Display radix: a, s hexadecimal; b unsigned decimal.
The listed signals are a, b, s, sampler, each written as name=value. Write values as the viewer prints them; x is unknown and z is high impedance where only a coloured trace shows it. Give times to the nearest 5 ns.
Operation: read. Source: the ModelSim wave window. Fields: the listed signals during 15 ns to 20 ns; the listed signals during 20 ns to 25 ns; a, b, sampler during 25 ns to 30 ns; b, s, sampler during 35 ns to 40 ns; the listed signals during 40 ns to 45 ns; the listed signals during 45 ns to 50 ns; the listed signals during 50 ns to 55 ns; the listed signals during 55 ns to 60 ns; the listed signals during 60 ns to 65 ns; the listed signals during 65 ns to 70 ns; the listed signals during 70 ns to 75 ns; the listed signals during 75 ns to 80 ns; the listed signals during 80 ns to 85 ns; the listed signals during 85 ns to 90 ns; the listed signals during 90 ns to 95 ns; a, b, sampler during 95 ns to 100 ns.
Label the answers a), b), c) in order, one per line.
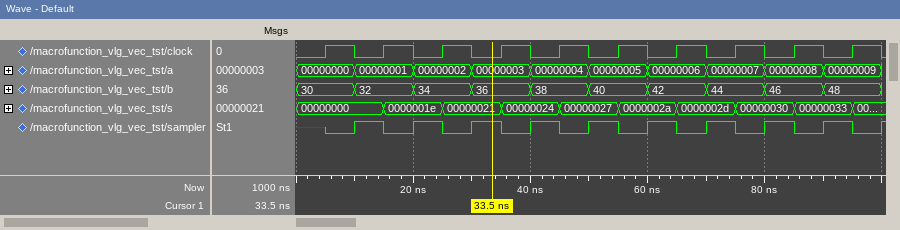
a) a=00000001, b=32, s=0000001e, sampler=0
b) a=00000002, b=34, s=0000001e, sampler=1
c) a=00000002, b=34, sampler=0
d) b=36, s=00000024, sampler=0
e) a=00000004, b=38, s=00000024, sampler=1
f) a=00000004, b=38, s=00000027, sampler=0
g) a=00000005, b=40, s=00000027, sampler=1
h) a=00000005, b=40, s=0000002a, sampler=0
i) a=00000006, b=42, s=0000002a, sampler=1
j) a=00000006, b=42, s=0000002d, sampler=0
k) a=00000007, b=44, s=0000002d, sampler=1
l) a=00000007, b=44, s=00000030, sampler=0
m) a=00000008, b=46, s=00000030, sampler=1
n) a=00000008, b=46, s=00000033, sampler=0
o) a=00000009, b=48, s=00000033, sampler=1
p) a=00000009, b=48, sampler=0
